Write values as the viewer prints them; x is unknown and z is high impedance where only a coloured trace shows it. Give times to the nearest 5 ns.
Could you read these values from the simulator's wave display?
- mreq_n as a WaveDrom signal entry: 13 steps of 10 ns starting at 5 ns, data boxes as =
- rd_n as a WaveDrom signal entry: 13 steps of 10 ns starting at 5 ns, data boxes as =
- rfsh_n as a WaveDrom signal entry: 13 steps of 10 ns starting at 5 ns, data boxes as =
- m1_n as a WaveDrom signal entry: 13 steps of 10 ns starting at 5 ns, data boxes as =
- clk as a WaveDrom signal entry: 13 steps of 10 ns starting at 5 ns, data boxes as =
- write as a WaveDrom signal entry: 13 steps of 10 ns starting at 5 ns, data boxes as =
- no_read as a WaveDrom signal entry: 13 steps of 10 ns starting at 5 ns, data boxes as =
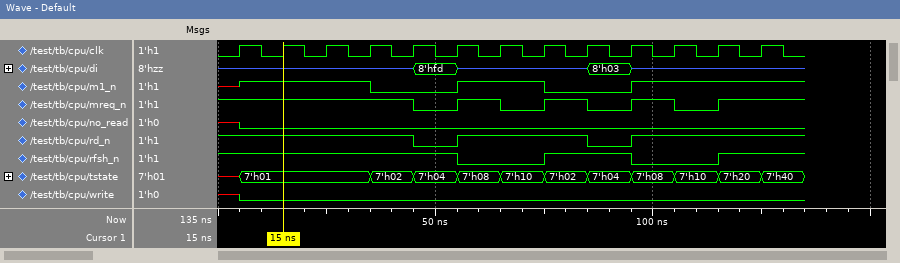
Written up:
{name: 'mreq_n', wave: '1...01010101.'}
{name: 'rd_n', wave: '1...01..01...'}
{name: 'rfsh_n', wave: '1....0.1.0.1.'}
{name: 'm1_n', wave: '1..0.1.0.1...'}
{name: 'clk', wave: 'p............'}
{name: 'write', wave: '0............'}
{name: 'no_read', wave: '0............'}
